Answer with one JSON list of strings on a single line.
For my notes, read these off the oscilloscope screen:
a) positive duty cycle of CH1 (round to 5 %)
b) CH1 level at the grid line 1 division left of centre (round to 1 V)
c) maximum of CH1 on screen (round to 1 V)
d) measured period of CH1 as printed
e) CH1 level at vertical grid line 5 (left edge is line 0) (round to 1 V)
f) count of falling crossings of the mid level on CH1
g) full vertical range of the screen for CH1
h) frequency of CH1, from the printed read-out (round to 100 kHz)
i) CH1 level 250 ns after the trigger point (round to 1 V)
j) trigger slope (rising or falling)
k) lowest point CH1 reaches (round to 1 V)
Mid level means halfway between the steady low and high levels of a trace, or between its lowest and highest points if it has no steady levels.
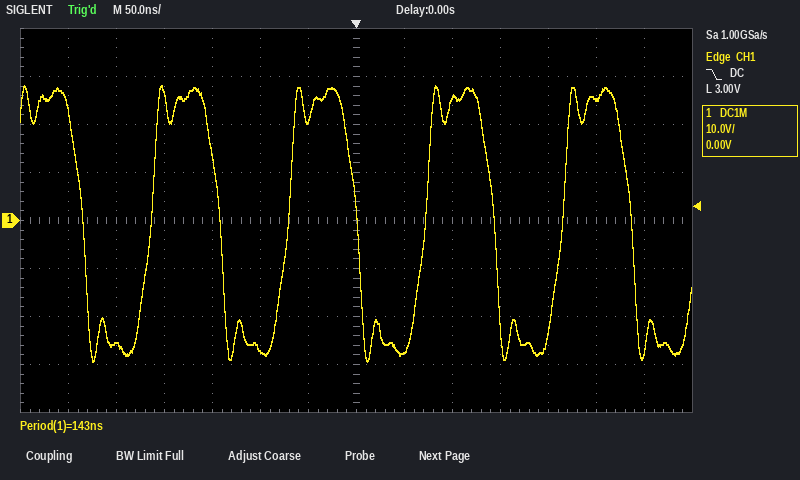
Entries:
["50 %", "21 V", "28 V", "143 ns", "-27 V", "5", "80 V", "7.0 MHz", "25 V", "falling", "-29 V"]
